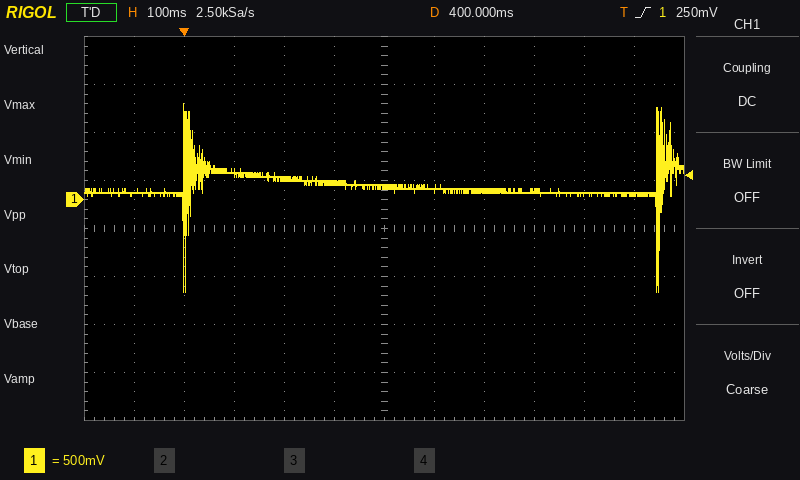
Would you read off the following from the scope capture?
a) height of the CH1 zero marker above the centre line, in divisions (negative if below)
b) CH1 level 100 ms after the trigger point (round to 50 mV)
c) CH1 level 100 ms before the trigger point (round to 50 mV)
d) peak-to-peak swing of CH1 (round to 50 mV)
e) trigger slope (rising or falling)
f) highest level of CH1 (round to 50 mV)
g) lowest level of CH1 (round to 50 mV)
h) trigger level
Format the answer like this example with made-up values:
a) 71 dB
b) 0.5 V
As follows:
a) +0.6 div
b) 300 mV
c) 50 mV
d) 1.95 V
e) rising
f) 1.00 V
g) -950 mV
h) 250 mV
